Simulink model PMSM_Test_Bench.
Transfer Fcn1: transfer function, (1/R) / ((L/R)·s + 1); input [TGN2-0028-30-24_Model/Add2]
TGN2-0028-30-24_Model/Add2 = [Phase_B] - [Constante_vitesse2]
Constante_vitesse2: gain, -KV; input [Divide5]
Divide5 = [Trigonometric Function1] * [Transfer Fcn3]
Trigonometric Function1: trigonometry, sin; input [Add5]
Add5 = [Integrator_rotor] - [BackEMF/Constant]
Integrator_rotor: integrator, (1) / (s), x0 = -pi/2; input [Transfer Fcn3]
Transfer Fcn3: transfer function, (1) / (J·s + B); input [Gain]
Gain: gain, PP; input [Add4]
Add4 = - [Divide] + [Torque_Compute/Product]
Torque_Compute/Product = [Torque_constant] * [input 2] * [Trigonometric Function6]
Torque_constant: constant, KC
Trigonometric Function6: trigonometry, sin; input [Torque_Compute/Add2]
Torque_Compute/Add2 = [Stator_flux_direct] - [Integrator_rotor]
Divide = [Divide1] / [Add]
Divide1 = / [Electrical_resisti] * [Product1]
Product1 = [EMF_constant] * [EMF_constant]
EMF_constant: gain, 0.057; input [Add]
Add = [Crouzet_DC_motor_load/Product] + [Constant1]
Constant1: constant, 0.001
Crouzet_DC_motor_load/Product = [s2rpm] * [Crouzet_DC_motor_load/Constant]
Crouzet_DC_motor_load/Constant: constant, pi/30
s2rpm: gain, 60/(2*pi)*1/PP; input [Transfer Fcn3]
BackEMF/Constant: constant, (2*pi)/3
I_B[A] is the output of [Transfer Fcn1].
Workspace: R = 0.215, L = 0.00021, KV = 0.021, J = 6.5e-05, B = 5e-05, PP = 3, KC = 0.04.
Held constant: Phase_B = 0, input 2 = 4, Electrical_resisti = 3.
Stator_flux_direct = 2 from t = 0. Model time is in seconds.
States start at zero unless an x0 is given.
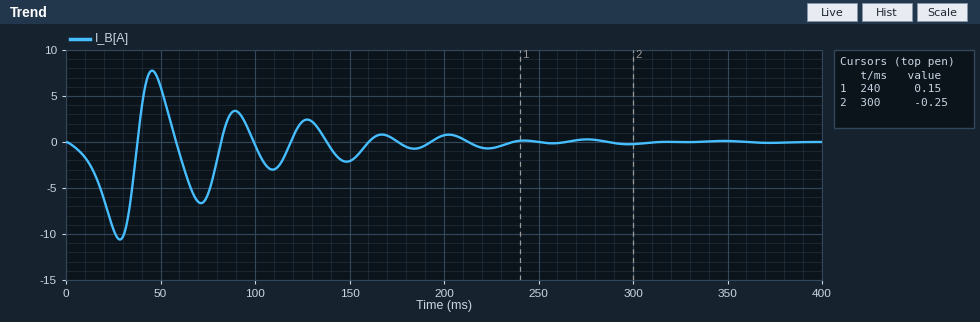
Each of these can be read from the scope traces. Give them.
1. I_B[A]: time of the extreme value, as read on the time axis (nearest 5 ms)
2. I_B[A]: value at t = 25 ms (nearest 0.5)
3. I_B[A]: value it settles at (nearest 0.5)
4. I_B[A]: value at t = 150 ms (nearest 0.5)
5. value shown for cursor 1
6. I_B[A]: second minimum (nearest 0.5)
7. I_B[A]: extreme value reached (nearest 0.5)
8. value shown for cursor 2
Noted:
30 ms
-9.5
0.0
-2.0
0.15
-6.5
-10.5
-0.25
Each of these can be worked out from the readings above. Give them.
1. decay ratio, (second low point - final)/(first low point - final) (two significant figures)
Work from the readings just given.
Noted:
0.62
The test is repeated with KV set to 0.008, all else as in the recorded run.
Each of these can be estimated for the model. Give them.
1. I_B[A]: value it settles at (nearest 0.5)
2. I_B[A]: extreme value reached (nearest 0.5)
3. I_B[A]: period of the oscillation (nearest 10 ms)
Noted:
0.0
-4.0
40 ms
